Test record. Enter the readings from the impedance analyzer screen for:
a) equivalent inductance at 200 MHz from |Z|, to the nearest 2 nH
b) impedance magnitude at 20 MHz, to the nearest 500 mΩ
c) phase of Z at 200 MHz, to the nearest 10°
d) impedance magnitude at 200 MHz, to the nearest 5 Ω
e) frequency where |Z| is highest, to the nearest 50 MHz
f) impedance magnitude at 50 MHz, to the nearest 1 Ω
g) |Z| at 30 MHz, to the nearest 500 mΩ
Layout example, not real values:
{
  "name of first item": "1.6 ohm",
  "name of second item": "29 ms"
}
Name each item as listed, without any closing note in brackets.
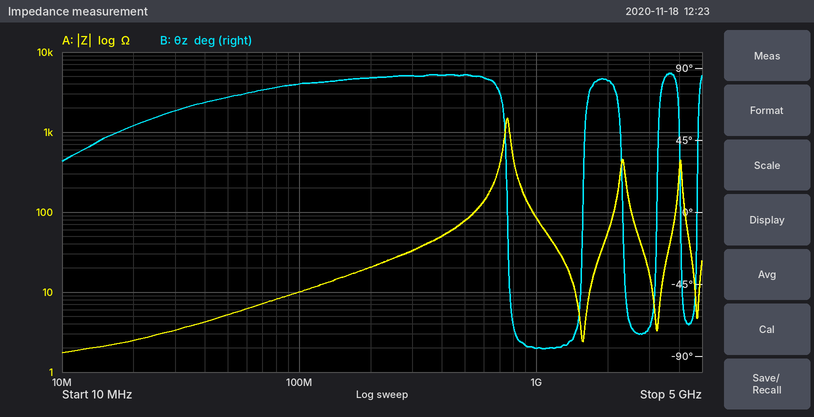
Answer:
{
  "equivalent inductance at 200 MHz from |Z|, to the nearest 2 nH": "16 nH",
  "impedance magnitude at 20 MHz, to the nearest 500 mΩ": "2.5 Ω",
  "phase of Z at 200 MHz, to the nearest 10°": "80°",
  "impedance magnitude at 200 MHz, to the nearest 5 Ω": "20 Ω",
  "frequency where |Z| is highest, to the nearest 50 MHz": "750 MHz",
  "impedance magnitude at 50 MHz, to the nearest 1 Ω": "5 Ω",
  "|Z| at 30 MHz, to the nearest 500 mΩ": "3.5 Ω"
}
